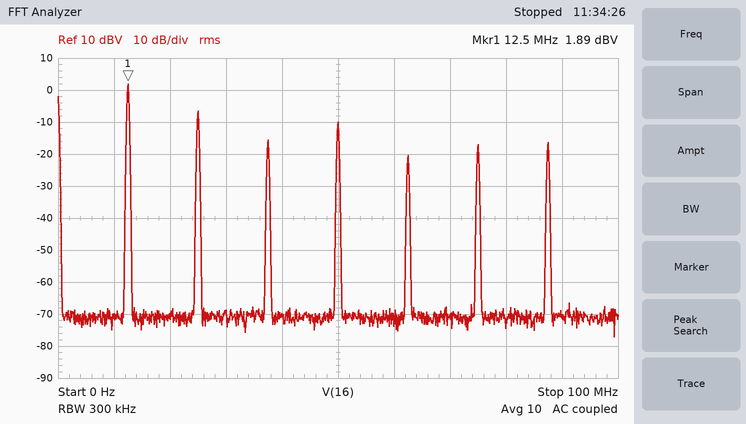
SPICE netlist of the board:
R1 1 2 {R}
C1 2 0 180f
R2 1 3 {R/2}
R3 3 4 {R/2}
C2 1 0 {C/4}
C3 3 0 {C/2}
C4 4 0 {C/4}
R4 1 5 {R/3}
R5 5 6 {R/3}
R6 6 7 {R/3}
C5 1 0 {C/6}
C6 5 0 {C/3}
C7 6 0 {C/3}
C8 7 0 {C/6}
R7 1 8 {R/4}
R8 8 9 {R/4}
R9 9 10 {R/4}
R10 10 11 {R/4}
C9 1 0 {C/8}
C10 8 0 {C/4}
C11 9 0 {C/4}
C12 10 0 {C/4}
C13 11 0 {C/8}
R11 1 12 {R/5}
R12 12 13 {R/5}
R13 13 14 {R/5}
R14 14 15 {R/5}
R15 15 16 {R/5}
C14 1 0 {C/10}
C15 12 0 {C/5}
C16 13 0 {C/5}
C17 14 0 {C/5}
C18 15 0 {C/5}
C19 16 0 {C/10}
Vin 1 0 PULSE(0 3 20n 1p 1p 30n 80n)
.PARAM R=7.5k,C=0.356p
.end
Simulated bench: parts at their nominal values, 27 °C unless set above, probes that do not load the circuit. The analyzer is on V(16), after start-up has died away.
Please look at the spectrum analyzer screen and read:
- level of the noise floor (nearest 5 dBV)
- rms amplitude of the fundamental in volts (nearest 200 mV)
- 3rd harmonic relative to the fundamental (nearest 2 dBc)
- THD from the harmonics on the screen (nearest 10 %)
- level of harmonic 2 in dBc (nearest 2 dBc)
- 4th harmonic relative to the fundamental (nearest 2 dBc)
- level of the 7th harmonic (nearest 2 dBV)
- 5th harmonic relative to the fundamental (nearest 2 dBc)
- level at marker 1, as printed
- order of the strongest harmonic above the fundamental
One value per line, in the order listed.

-70 dBV
1.2 V
-18 dBc
50 %
-8 dBc
-12 dBc
-16 dBV
-22 dBc
1.89 dBV
2
